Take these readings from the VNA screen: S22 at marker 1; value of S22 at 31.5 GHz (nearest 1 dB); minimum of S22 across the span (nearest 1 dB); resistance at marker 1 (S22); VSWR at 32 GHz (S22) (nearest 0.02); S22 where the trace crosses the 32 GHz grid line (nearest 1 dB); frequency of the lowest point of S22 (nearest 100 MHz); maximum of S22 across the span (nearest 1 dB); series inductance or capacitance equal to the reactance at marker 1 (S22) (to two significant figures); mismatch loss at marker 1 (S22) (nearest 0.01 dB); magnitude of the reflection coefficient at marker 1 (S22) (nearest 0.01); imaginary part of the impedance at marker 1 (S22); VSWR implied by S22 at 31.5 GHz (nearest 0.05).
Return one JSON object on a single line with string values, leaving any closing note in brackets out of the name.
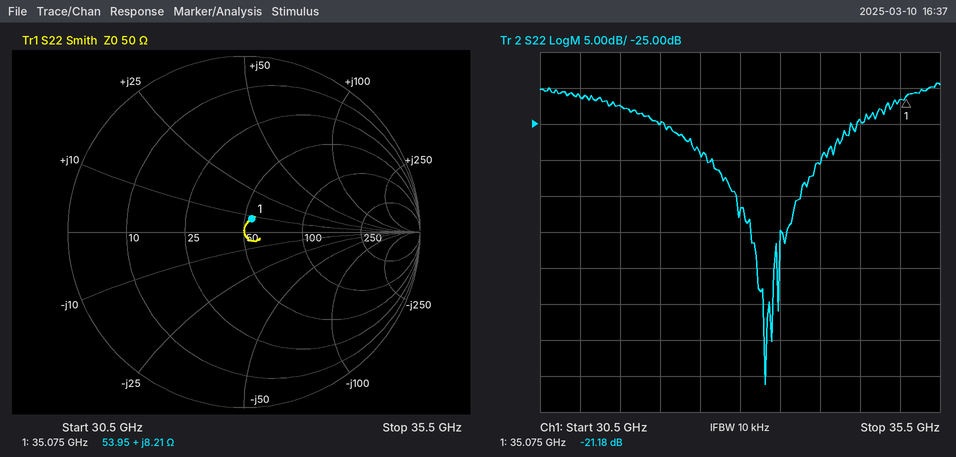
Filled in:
{"S22 at marker 1": "-21.18 dB", "value of S22 at 31.5 GHz": "-22 dB", "minimum of S22 across the span": "-61 dB", "resistance at marker 1": "53.95 Ω", "VSWR at 32 GHz (S22)": "1.12", "S22 where the trace crosses the 32 GHz grid line": "-25 dB", "frequency of the lowest point of S22": "33.3 GHz", "maximum of S22 across the span": "-19 dB", "series inductance or capacitance equal to the reactance at marker 1 (S22)": "37 pH", "mismatch loss at marker 1 (S22)": "0.03 dB", "magnitude of the reflection coefficient at marker 1 (S22)": "0.09", "imaginary part of the impedance at marker 1": "+8.21 Ω", "VSWR implied by S22 at 31.5 GHz": "1.15"}
